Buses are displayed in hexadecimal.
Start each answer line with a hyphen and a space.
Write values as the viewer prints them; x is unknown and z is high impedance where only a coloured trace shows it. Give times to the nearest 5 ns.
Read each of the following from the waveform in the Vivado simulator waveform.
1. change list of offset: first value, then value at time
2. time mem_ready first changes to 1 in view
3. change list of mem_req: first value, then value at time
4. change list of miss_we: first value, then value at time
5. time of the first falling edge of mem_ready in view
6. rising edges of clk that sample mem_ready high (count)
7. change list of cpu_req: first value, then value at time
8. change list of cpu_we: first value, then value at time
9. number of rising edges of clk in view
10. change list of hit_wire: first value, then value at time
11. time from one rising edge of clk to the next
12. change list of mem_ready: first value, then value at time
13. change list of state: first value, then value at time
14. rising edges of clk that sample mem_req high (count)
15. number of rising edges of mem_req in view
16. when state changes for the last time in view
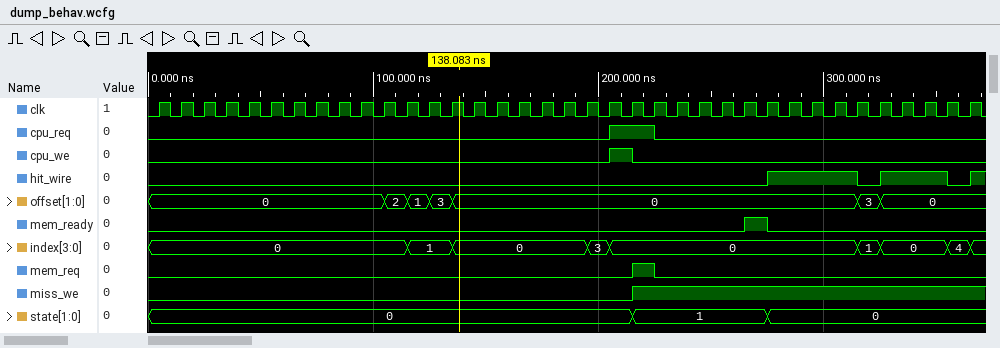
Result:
- 0, 2 at 105 ns, 1 at 115 ns, 3 at 125 ns, 0 at 135 ns, 3 at 315 ns, 0 at 325 ns
- 265 ns
- 0, 1 at 215 ns, 0 at 225 ns
- 0, 1 at 215 ns
- 275 ns
- 1
- 0, 1 at 205 ns, 0 at 225 ns
- 0, 1 at 205 ns, 0 at 215 ns
- 37
- 0, 1 at 275 ns, 0 at 315 ns, 1 at 325 ns, 0 at 355 ns, 1 at 365 ns
- 10 ns
- 0, 1 at 265 ns, 0 at 275 ns
- 0, 1 at 215 ns, 0 at 275 ns
- 1
- 1
- 275 ns
